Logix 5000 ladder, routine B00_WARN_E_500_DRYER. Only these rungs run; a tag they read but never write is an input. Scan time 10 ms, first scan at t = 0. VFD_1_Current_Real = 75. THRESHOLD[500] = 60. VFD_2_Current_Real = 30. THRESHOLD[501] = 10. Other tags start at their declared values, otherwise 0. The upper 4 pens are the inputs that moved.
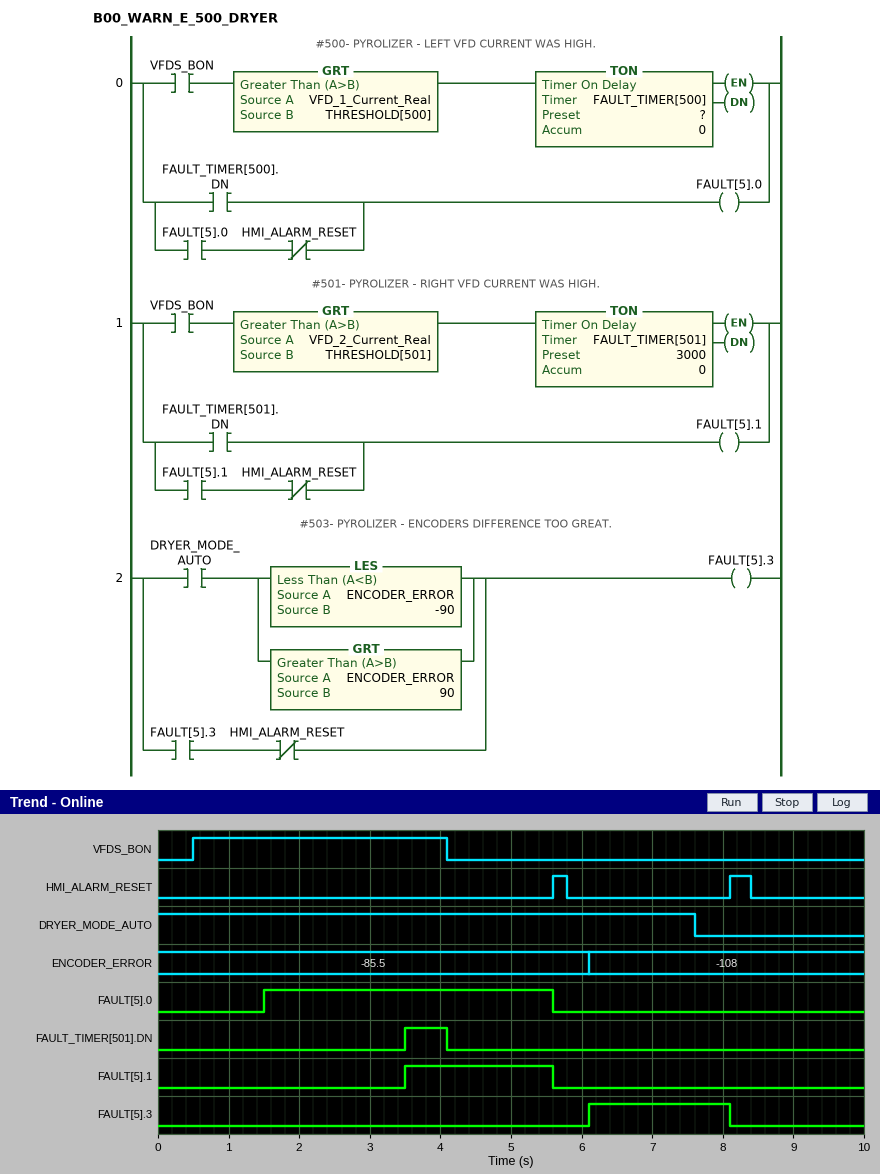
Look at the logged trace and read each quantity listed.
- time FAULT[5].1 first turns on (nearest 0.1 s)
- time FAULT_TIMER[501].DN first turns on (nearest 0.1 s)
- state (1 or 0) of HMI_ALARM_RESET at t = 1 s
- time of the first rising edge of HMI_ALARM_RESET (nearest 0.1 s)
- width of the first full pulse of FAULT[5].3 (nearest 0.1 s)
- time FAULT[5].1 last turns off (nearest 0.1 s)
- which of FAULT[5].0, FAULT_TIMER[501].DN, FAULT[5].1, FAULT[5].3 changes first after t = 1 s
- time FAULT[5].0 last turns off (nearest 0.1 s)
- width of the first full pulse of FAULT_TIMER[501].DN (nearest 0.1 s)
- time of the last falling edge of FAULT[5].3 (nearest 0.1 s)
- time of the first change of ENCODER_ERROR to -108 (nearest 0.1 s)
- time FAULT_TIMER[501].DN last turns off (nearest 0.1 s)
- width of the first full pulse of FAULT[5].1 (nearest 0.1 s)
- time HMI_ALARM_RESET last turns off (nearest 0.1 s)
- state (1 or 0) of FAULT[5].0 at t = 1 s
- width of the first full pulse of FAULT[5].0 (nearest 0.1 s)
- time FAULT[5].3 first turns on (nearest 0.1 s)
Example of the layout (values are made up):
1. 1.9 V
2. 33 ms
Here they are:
1. 3.5 s
2. 3.5 s
3. 0
4. 5.6 s
5. 2.0 s
6. 5.6 s
7. FAULT[5].0
8. 5.6 s
9. 0.6 s
10. 8.1 s
11. 6.1 s
12. 4.1 s
13. 2.1 s
14. 8.4 s
15. 0
16. 4.1 s
17. 6.1 s
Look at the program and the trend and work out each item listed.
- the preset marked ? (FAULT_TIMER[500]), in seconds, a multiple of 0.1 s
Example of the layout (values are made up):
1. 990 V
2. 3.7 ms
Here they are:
1. 1.0 s
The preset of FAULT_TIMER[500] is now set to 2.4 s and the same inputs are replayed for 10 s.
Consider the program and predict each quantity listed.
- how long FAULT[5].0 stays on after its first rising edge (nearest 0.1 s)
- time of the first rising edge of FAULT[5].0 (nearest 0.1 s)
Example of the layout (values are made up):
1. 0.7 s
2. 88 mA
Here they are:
1. 2.7 s
2. 2.9 s
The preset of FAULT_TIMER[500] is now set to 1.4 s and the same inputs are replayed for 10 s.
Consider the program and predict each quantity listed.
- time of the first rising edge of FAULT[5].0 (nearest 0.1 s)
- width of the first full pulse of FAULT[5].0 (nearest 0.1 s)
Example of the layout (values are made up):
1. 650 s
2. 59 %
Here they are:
1. 1.9 s
2. 3.7 s
